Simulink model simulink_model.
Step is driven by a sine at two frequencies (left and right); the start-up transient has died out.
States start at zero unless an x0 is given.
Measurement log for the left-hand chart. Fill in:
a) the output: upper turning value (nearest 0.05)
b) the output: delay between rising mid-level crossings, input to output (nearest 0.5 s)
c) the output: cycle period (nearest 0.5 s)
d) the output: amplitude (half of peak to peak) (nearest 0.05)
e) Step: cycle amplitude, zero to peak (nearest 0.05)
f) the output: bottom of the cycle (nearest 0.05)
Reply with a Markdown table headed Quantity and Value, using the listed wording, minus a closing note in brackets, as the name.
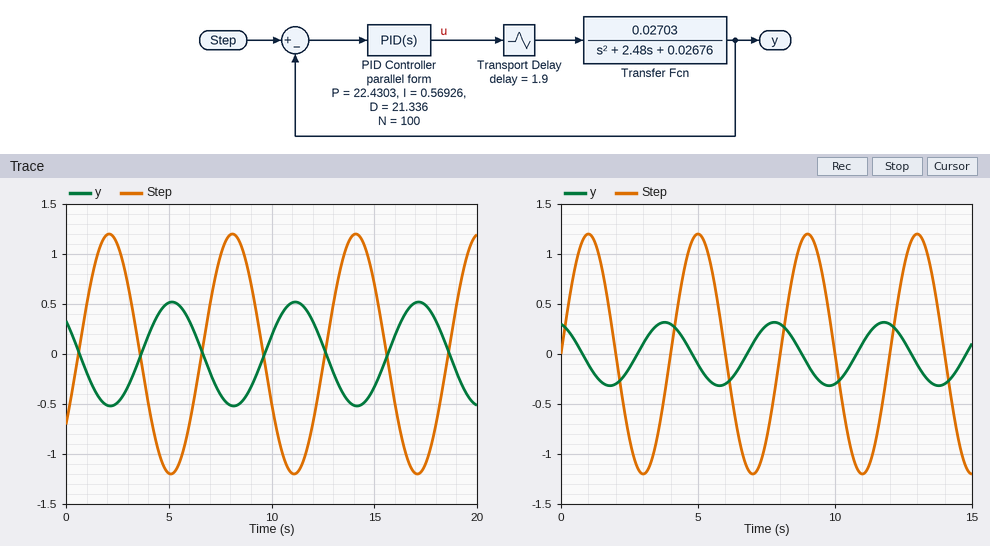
| Quantity | Value |
|---|---|
| the output: upper turning value | 0.50 |
| the output: delay between rising mid-level crossings, input to output | 3.0 s |
| the output: cycle period | 6.0 s |
| the output: amplitude (half of peak to peak) | 0.50 |
| Step: cycle amplitude, zero to peak | 1.20 |
| the output: bottom of the cycle | -0.50 |
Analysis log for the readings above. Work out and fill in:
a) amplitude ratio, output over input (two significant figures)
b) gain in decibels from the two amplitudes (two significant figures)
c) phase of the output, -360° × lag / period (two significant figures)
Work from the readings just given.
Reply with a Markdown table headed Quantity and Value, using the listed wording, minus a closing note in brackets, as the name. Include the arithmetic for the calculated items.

| Quantity | Value |
|---|---|
| amplitude ratio, output over input | 0.5 / 1.2 = 0.42 |
| gain in decibels from the two amplitudes | 20 log10(0.5 / 1.2) = -7.6 dB |
| phase of the output, -360° × lag / period | -360 × 3 / 6 = -180° |
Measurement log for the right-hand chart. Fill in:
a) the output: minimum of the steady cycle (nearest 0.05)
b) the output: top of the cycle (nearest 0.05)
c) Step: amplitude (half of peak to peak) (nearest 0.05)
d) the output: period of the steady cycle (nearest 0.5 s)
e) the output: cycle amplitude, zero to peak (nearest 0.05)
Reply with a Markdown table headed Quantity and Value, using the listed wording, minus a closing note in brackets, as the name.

| Quantity | Value |
|---|---|
| the output: minimum of the steady cycle | -0.30 |
| the output: top of the cycle | 0.30 |
| Step: amplitude (half of peak to peak) | 1.20 |
| the output: period of the steady cycle | 4.0 s |
| the output: cycle amplitude, zero to peak | 0.30 |
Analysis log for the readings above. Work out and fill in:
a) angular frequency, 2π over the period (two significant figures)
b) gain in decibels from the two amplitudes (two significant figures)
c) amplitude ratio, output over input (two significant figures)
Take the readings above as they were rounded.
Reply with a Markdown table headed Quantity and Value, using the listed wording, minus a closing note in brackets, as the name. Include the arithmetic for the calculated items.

| Quantity | Value |
|---|---|
| angular frequency, 2π over the period | 2π / 4 = 1.6 rad/s |
| gain in decibels from the two amplitudes | 20 log10(0.3 / 1.2) = -12 dB |
| amplitude ratio, output over input | 0.3 / 1.2 = 0.25 |
